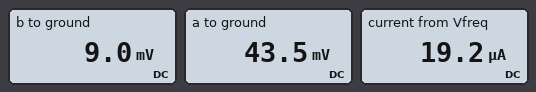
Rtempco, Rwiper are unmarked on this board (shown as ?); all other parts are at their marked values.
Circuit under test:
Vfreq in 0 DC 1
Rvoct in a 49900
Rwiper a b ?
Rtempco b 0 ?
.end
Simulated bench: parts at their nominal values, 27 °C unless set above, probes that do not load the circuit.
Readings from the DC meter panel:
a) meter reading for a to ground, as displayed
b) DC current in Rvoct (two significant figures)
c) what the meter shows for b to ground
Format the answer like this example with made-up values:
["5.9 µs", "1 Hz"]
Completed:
["43.5 mV", "19 µA", "9.0 mV"]
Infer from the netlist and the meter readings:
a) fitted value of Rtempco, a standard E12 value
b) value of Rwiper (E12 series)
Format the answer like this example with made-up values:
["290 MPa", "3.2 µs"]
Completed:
["470 Ω", "1.8 kΩ"]
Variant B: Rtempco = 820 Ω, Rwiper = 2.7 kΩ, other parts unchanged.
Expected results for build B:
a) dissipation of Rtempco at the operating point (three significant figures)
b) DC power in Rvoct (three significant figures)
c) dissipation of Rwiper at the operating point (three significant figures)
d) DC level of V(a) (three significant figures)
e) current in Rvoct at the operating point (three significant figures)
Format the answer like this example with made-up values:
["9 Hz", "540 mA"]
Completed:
["287 nW", "17.5 µW", "946 nW", "65.9 mV", "18.7 µA"]
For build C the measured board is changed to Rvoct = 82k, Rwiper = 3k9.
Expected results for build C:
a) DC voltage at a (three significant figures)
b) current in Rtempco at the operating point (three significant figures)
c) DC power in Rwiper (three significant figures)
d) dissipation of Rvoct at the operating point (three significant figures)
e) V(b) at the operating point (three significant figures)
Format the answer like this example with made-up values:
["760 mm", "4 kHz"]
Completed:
["50.6 mV", "11.6 µA", "523 nW", "11.0 µW", "5.44 mV"]
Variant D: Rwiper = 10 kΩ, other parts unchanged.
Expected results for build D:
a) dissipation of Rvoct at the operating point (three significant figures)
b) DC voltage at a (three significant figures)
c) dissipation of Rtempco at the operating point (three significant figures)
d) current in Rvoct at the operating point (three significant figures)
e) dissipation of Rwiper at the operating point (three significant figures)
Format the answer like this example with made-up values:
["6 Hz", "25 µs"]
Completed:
["13.7 µW", "173 mV", "129 nW", "16.6 µA", "2.74 µW"]
